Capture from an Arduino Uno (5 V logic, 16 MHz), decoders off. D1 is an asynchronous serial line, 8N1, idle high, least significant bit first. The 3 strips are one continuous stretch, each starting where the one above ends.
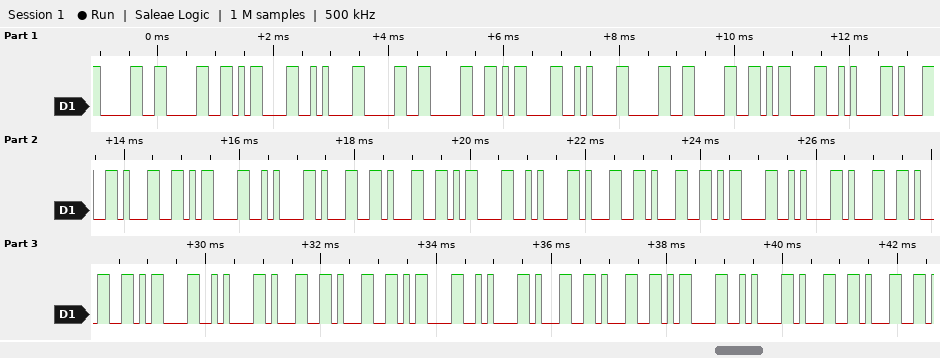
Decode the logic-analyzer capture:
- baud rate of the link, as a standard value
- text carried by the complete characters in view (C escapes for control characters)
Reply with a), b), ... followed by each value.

a) 9600 baud
b) "00\r\n00\r\n00\r\n11\r\n11\r\n11\r\n11\r\n11\r\n11\r\n11"
